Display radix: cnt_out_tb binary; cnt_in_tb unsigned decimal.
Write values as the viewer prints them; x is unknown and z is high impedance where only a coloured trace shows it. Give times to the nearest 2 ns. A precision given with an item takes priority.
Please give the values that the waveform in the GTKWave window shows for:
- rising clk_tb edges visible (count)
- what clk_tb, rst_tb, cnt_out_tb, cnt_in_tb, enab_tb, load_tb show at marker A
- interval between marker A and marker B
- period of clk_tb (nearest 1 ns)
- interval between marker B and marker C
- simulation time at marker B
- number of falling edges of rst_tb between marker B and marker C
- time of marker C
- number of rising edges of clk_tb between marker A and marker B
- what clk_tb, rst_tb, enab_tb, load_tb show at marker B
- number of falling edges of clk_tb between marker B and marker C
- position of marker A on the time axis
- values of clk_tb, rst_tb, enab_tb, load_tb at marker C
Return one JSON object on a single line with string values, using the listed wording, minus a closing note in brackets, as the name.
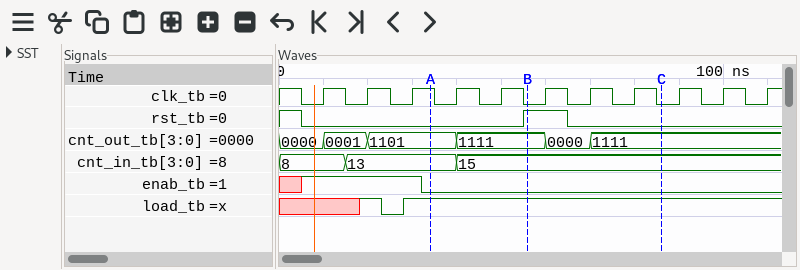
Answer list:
{"rising clk_tb edges visible": "11", "what clk_tb, rst_tb, cnt_out_tb, cnt_in_tb, enab_tb, load_tb show at marker A": "clk_tb=1, rst_tb=0, cnt_out_tb=1101, cnt_in_tb=13, enab_tb=0, load_tb=1", "interval between marker A and marker B": "22 ns", "period of clk_tb": "10 ns", "interval between marker B and marker C": "30 ns", "simulation time at marker B": "56 ns", "number of falling edges of rst_tb between marker B and marker C": "1", "time of marker C": "86 ns", "number of rising edges of clk_tb between marker A and marker B": "2", "what clk_tb, rst_tb, enab_tb, load_tb show at marker B": "clk_tb=0, rst_tb=1, enab_tb=0, load_tb=1", "number of falling edges of clk_tb between marker B and marker C": "3", "position of marker A on the time axis": "34 ns", "values of clk_tb, rst_tb, enab_tb, load_tb at marker C": "clk_tb=0, rst_tb=0, enab_tb=0, load_tb=1"}
